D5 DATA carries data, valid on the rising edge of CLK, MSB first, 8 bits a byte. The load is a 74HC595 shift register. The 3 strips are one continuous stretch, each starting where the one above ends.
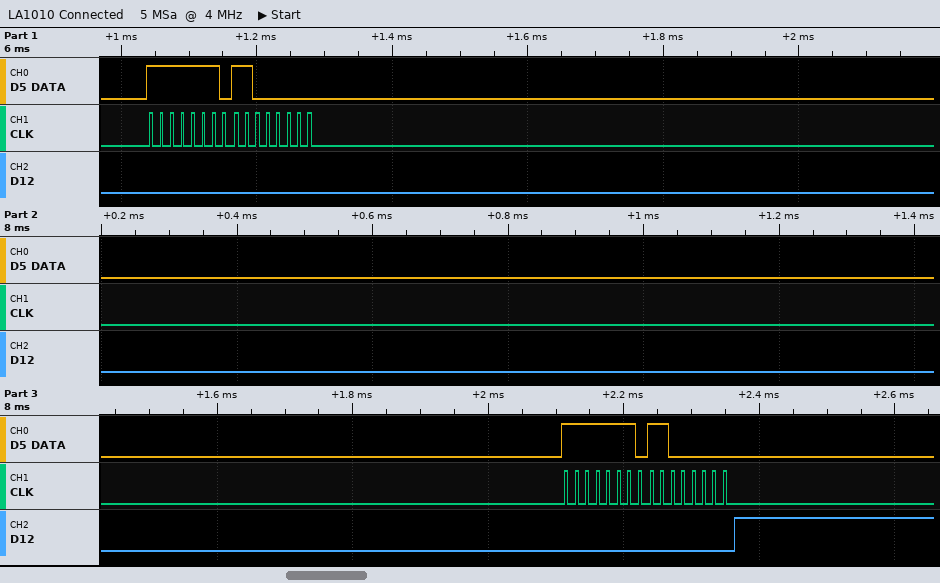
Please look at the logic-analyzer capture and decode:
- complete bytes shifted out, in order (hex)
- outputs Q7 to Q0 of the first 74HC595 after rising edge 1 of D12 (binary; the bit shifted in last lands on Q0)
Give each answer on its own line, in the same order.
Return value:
FE C0 FE C0
11000000
